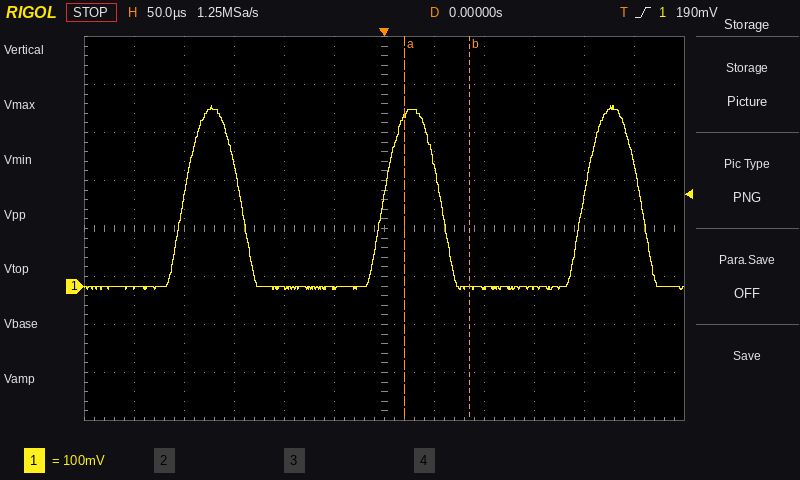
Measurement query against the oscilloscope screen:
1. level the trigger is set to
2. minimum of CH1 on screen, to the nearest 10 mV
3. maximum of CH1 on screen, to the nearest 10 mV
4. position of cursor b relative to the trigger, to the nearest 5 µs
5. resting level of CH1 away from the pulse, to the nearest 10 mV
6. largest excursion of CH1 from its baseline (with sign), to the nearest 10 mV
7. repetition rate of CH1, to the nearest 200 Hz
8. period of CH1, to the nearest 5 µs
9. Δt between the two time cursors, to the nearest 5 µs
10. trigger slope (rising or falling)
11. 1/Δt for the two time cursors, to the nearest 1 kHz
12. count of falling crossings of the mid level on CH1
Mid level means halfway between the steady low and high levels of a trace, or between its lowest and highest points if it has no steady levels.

190 mV
-10 mV
380 mV
+85 µs
0 mV
+380 mV
5.0 kHz
200 µs
65 µs
rising
15 kHz
3
